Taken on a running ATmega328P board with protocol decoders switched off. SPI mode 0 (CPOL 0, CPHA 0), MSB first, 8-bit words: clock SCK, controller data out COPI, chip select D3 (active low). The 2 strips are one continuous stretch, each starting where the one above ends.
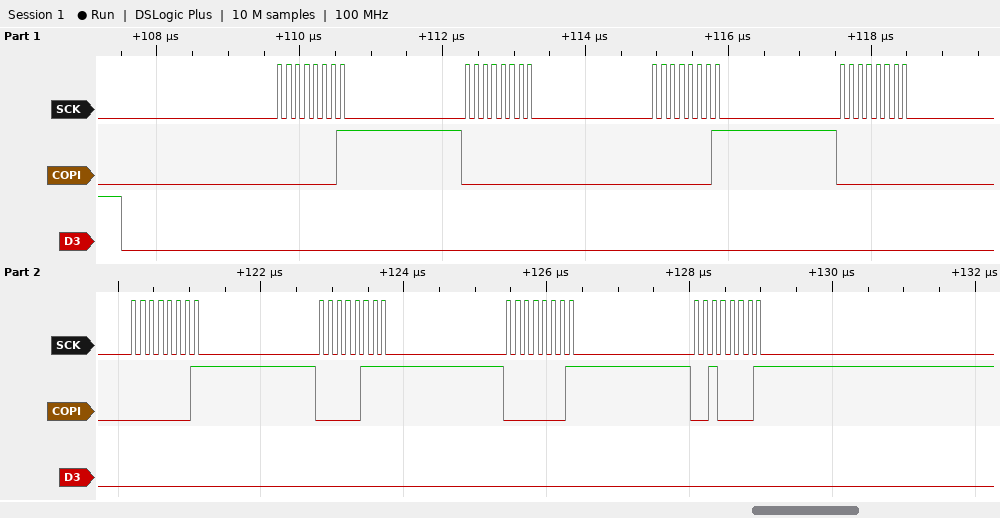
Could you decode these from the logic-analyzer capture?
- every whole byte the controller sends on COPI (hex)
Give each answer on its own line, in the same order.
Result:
0x01 0x00 0x01 0x00 0x01 0x07 0x01 0x21
